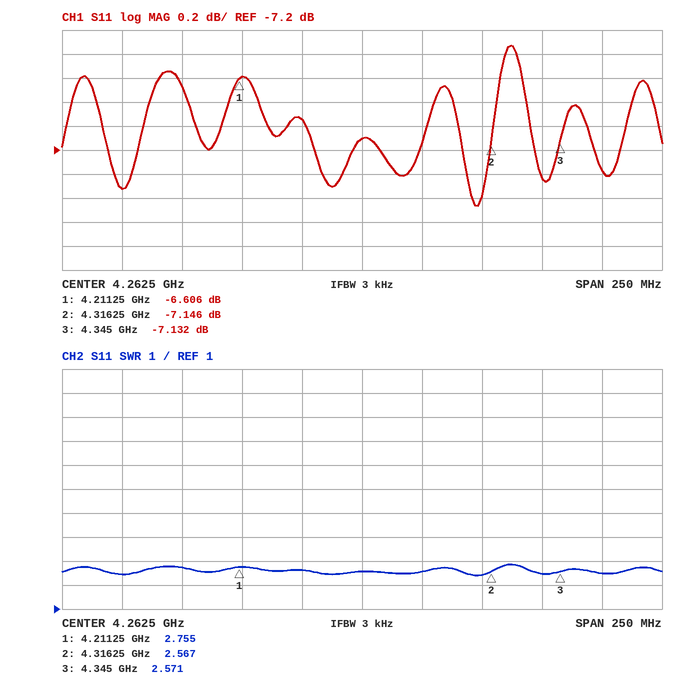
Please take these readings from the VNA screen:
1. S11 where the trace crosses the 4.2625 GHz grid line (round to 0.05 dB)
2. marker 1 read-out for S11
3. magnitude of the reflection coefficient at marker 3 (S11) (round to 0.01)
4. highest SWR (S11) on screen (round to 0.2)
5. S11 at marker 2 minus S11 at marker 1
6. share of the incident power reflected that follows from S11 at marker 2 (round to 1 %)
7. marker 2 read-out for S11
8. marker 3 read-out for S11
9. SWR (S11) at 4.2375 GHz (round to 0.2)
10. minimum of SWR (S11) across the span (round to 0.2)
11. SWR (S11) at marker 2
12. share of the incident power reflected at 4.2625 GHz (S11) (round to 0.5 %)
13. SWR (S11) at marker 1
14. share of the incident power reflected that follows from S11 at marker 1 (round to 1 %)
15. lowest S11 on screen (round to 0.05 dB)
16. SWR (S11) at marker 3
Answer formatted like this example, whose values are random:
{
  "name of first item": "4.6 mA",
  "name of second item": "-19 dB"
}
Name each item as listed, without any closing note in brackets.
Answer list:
{
  "S11 where the trace crosses the 4.2625 GHz grid line": "-7.10 dB",
  "marker 1 read-out for S11": "-6.606 dB",
  "magnitude of the reflection coefficient at marker 3 (S11)": "0.44",
  "highest SWR (S11) on screen": "2.8",
  "S11 at marker 2 minus S11 at marker 1": "-0.540 dB",
  "share of the incident power reflected that follows from S11 at marker 2": "19 %",
  "marker 2 read-out for S11": "-7.146 dB",
  "marker 3 read-out for S11": "-7.132 dB",
  "SWR (S11) at 4.2375 GHz": "2.6",
  "minimum of SWR (S11) across the span": "2.4",
  "SWR (S11) at marker 2": "2.567",
  "share of the incident power reflected at 4.2625 GHz (S11)": "19.5 %",
  "SWR (S11) at marker 1": "2.755",
  "share of the incident power reflected that follows from S11 at marker 1": "22 %",
  "lowest S11 on screen": "-7.65 dB",
  "SWR (S11) at marker 3": "2.571"
}
